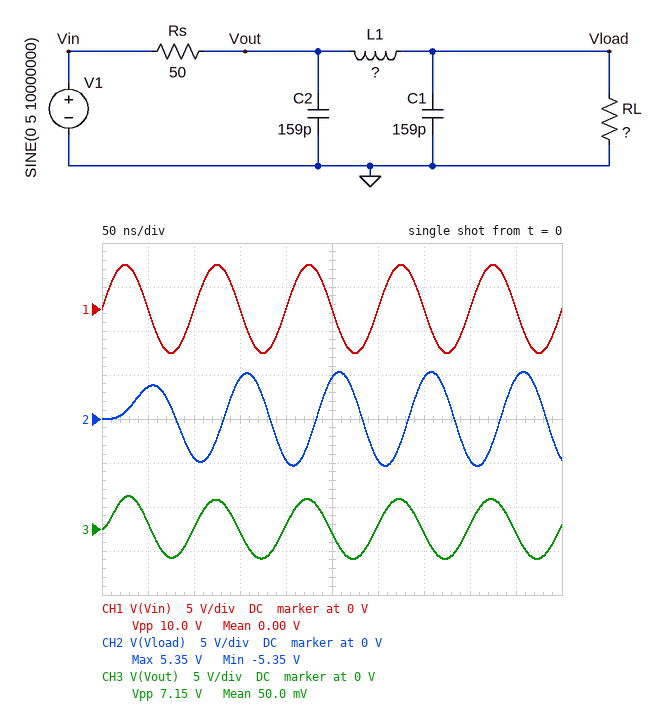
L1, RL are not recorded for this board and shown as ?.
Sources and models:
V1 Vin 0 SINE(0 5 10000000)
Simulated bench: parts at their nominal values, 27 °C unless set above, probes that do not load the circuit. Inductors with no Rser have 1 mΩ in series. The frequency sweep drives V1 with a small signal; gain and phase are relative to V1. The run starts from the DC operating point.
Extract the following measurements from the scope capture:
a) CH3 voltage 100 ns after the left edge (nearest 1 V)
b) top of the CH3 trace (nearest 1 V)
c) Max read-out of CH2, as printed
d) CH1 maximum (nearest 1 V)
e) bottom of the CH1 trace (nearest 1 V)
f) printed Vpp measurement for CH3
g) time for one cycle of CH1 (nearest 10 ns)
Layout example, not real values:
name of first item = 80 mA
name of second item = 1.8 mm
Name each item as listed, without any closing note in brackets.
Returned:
CH3 voltage 100 ns after the left edge = 0 V
top of the CH3 trace = 4 V
Max read-out of CH2, as printed = 5.35 V
CH1 maximum = 5 V
bottom of the CH1 trace = -5 V
printed Vpp measurement for CH3 = 7.15 V
time for one cycle of CH1 = 100 ns
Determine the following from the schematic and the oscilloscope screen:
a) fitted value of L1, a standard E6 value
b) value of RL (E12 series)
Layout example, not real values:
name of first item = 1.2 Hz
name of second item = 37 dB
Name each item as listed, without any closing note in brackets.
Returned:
fitted value of L1, a standard E6 value = 2.2 µH
value of RL = 270 Ω
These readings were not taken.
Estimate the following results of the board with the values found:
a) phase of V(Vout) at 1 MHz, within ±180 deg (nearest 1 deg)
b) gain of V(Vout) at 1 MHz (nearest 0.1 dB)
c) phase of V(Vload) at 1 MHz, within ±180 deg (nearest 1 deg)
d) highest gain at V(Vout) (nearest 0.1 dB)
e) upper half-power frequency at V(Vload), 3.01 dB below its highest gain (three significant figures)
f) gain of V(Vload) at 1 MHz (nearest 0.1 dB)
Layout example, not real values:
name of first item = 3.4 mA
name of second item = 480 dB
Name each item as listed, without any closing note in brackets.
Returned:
phase of V(Vout) at 1 MHz, within ±180 deg = -4 deg
gain of V(Vout) at 1 MHz = -1.5 dB
phase of V(Vload) at 1 MHz, within ±180 deg = -7 deg
highest gain at V(Vout) = -0.8 dB
upper half-power frequency at V(Vload), 3.01 dB below its highest gain = 11.6 MHz
gain of V(Vload) at 1 MHz = -1.4 dB
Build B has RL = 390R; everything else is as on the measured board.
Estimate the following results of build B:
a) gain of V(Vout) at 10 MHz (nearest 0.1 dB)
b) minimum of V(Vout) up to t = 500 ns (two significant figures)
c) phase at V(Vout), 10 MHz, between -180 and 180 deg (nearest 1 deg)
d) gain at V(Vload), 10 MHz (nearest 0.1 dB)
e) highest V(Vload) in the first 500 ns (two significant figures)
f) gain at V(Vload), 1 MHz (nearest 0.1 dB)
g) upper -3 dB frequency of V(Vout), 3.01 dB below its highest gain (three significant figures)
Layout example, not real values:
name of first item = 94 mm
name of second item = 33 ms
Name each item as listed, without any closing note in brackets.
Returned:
gain of V(Vout) at 10 MHz = -3.6 dB
minimum of V(Vout) up to t = 500 ns = -3.3 V
phase at V(Vout), 10 MHz, between -180 and 180 deg = 14 deg
gain at V(Vload), 10 MHz = 2.0 dB
highest V(Vload) in the first 500 ns = 6.3 V
gain at V(Vload), 1 MHz = -1.0 dB
upper -3 dB frequency of V(Vout), 3.01 dB below its highest gain = 26.1 MHz
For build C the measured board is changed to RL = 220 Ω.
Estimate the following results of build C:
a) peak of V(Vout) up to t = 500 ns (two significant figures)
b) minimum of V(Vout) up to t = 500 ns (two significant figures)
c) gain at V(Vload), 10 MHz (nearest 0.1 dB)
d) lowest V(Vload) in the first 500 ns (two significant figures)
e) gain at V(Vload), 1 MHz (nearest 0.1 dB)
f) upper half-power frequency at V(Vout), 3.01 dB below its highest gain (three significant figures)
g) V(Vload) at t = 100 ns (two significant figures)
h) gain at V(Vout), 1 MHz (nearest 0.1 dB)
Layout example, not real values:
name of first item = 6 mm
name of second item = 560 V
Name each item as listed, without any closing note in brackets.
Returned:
peak of V(Vout) up to t = 500 ns = 3.7 V
minimum of V(Vout) up to t = 500 ns = -3.5 V
gain at V(Vload), 10 MHz = -0.4 dB
lowest V(Vload) in the first 500 ns = -4.8 V
gain at V(Vload), 1 MHz = -1.7 dB
upper half-power frequency at V(Vout), 3.01 dB below its highest gain = 27.1 MHz
V(Vload) at t = 100 ns = -4.1 V
gain at V(Vout), 1 MHz = -1.8 dB
